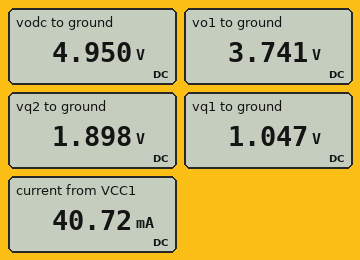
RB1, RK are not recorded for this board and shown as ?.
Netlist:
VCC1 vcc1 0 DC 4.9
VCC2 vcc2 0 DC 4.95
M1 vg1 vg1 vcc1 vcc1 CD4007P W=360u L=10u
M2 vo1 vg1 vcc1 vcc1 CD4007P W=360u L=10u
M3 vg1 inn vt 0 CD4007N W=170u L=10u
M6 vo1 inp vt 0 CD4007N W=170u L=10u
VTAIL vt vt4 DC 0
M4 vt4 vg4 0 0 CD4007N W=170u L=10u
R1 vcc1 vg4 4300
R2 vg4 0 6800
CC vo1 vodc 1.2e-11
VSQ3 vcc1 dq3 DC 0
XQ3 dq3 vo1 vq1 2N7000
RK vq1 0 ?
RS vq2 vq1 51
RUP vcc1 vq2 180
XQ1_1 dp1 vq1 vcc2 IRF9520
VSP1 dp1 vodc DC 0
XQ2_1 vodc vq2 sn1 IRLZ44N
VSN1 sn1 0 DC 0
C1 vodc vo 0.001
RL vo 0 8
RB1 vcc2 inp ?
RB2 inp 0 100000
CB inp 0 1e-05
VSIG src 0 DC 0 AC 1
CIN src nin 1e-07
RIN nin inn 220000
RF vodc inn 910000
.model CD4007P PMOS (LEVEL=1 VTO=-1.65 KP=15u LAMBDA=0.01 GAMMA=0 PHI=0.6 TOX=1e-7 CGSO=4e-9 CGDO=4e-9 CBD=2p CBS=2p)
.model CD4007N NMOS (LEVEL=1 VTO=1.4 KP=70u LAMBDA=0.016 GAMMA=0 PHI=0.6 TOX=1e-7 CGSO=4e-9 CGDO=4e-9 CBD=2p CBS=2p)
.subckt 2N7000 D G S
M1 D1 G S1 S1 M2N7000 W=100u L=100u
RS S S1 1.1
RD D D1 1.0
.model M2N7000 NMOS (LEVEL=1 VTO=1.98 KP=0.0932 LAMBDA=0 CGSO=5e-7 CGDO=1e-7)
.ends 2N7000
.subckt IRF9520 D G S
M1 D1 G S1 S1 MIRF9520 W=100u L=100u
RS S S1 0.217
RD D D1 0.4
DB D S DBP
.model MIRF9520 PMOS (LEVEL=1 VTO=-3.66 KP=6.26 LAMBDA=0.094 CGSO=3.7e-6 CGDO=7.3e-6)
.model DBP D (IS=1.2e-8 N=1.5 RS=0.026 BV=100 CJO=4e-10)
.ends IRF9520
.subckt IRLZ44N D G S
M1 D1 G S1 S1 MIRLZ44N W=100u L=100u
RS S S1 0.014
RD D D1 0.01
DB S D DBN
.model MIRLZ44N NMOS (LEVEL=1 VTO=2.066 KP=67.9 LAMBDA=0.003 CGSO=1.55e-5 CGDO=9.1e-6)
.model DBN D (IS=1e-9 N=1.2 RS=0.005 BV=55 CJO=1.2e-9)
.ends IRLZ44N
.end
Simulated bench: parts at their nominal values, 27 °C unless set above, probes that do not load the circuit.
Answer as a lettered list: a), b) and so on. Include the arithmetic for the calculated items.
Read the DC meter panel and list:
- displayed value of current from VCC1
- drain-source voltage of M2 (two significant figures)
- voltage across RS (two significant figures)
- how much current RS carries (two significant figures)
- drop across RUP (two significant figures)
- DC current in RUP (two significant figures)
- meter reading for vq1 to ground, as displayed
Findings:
a) 40.72 mA
b) 3.741 V - 4.9 V = -1.2 V
c) 1.898 V - 1.047 V = 850 mV
d) (1.898 V - 1.047 V) / 51 Ω = 17 mA
e) 4.9 V - 1.898 V = 3.0 V
f) (4.9 V - 1.898 V) / 180 Ω = 17 mA
g) 1.047 V
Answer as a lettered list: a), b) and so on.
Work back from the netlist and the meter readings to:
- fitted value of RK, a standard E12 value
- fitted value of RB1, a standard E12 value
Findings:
a) 27 Ω
b) 33 kΩ
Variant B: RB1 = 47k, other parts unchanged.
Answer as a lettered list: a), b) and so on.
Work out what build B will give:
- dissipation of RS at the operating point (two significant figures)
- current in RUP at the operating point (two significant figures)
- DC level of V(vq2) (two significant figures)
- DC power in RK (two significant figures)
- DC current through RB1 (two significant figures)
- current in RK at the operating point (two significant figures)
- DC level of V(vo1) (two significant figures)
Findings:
a) 13 mW
b) 16 mA
c) 2.1 V
d) 60 mW
e) 34 µA
f) 47 mA
g) 4.1 V
